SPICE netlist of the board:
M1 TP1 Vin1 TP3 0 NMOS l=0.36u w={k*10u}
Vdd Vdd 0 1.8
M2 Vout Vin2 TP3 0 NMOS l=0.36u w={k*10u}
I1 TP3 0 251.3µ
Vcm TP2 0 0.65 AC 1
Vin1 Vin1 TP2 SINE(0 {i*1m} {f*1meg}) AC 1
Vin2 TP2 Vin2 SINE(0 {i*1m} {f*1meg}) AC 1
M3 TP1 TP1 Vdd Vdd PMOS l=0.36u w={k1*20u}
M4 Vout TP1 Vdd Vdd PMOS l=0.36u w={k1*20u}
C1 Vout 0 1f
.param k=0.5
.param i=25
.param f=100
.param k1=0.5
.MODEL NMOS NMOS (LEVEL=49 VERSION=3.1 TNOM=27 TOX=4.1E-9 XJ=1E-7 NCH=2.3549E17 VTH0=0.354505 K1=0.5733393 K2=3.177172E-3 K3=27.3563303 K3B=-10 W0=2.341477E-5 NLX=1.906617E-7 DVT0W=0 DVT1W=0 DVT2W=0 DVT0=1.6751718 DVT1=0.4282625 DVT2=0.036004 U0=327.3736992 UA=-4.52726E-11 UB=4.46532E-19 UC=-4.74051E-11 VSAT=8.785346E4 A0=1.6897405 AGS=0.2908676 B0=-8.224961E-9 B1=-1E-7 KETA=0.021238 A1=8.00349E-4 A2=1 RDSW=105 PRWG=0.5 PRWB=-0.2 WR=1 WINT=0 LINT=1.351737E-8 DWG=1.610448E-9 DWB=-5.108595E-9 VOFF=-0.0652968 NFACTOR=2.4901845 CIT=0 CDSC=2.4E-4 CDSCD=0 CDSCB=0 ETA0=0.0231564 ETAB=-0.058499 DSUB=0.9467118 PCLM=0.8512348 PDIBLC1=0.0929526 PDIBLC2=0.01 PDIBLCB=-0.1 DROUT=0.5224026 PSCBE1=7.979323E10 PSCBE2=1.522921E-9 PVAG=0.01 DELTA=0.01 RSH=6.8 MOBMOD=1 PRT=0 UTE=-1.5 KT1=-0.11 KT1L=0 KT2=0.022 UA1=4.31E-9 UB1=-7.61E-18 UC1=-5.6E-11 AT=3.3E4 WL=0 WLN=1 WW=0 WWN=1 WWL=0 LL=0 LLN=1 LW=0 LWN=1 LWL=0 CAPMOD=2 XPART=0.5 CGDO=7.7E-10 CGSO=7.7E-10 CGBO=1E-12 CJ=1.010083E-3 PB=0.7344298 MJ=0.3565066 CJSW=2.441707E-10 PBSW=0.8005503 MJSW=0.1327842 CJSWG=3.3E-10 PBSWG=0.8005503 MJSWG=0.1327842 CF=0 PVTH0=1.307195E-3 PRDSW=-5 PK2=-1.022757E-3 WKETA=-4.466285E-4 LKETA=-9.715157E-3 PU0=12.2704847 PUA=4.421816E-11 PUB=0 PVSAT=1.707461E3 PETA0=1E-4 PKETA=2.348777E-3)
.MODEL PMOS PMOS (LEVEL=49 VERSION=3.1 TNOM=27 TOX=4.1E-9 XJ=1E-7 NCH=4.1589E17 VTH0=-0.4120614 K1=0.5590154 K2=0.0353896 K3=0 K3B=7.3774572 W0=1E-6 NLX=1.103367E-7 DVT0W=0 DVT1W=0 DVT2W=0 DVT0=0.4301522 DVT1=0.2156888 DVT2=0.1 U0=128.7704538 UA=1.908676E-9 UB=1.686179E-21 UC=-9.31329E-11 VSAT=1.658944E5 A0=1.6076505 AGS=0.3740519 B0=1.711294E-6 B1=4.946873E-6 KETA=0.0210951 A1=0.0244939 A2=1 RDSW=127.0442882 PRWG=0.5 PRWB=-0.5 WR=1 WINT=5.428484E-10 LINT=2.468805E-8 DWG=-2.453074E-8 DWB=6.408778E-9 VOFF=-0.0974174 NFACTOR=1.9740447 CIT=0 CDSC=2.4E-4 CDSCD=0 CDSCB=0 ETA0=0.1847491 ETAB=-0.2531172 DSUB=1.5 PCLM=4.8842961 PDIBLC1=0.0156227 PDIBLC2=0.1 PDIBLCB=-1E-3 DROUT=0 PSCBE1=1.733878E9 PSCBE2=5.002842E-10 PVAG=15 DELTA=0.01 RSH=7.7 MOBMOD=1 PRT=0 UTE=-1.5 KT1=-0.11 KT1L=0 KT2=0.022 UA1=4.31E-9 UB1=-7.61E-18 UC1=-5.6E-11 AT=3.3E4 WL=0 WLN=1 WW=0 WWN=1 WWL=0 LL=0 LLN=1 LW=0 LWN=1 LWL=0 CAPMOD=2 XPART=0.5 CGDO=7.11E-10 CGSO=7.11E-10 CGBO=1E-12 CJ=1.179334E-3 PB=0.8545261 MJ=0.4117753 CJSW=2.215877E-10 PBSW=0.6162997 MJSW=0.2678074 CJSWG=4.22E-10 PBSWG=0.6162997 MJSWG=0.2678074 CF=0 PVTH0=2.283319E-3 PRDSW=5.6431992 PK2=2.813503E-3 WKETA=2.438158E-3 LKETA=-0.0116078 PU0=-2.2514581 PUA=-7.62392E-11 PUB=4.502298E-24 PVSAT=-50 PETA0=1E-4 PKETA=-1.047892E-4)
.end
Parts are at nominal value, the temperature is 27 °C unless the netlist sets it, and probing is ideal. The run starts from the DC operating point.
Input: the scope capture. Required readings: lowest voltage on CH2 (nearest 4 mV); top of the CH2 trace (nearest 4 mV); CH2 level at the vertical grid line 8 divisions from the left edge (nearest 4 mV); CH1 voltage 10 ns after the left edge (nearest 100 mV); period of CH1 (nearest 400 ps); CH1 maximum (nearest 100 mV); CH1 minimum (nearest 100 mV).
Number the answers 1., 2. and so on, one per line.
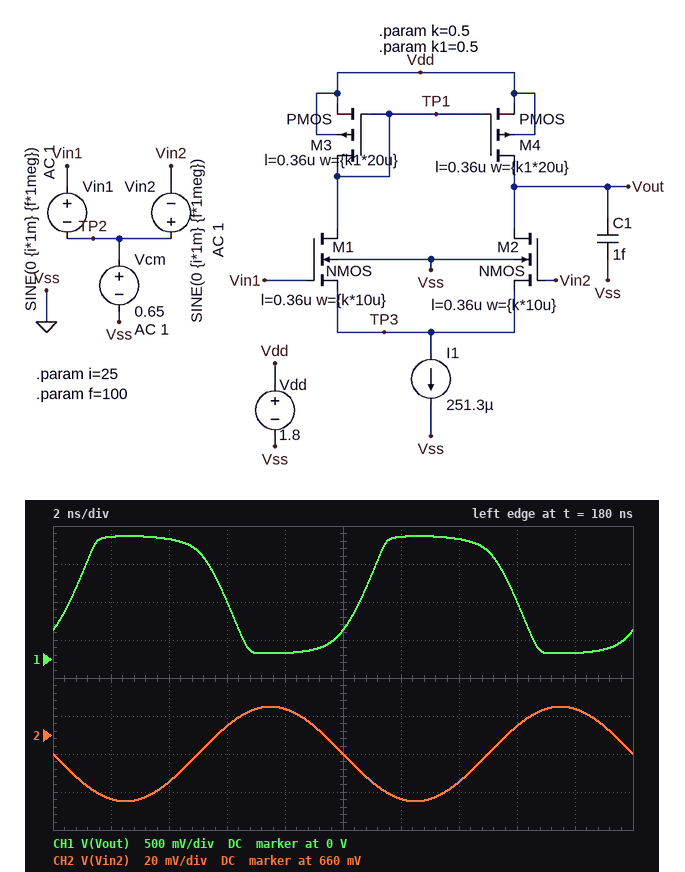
1. 624 mV
2. 676 mV
3. 664 mV
4. 400 mV
5. 10.0 ns
6. 1.6 V
7. 100 mV
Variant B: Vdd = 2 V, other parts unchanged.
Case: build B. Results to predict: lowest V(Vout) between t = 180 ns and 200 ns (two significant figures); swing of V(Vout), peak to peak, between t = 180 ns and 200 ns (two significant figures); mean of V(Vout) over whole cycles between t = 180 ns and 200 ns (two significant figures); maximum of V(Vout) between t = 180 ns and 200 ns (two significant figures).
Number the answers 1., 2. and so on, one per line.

1. 86 mV
2. 1.7 V
3. 1.0 V
4. 1.8 V
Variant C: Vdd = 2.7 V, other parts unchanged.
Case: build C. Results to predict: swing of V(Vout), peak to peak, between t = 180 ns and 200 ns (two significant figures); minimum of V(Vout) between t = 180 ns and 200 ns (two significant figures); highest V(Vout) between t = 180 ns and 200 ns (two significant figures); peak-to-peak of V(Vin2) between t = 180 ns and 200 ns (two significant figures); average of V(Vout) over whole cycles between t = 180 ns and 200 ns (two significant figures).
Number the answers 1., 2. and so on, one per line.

1. 2.4 V
2. 150 mV
3. 2.5 V
4. 50 mV
5. 1.5 V
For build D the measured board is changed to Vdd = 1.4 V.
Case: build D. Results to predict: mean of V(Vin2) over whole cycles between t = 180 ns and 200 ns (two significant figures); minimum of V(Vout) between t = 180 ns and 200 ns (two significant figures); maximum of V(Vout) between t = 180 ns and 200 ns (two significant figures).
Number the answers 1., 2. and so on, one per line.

1. 650 mV
2. 55 mV
3. 1.2 V
